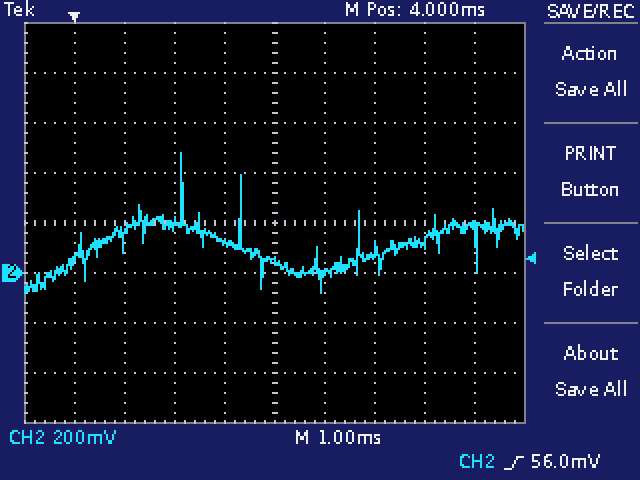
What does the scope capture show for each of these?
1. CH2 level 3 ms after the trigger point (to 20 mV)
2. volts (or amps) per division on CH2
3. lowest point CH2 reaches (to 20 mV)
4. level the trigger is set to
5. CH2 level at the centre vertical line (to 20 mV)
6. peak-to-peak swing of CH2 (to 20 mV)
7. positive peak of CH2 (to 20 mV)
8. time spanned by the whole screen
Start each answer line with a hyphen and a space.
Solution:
- 120 mV
- 200 mV
- -80 mV
- 56.0 mV
- 40 mV
- 560 mV
- 480 mV
- 10 ms
